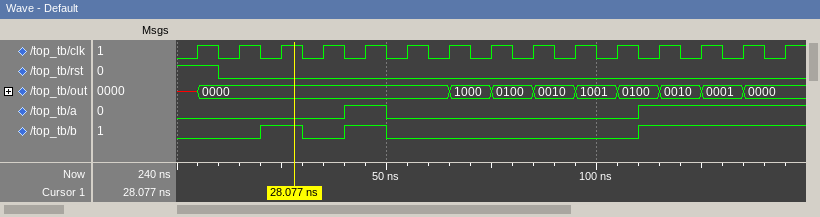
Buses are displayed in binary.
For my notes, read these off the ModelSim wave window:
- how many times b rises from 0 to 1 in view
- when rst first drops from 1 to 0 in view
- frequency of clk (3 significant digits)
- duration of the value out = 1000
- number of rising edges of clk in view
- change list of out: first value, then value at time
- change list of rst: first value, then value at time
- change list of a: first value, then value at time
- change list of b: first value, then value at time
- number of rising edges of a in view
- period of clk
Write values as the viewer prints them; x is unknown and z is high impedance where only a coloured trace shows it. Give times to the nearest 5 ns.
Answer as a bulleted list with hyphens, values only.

- 3
- 10 ns
- 100 MHz
- 10 ns
- 15
- x, 0000 at 5 ns, 1000 at 65 ns, 0100 at 75 ns, 0010 at 85 ns, 1001 at 95 ns, 0100 at 105 ns, 0010 at 115 ns, 0001 at 125 ns, 0000 at 135 ns
- 1, 0 at 10 ns
- 0, 1 at 40 ns, 0 at 50 ns, 1 at 110 ns
- 0, 1 at 20 ns, 0 at 30 ns, 1 at 40 ns, 0 at 50 ns, 1 at 110 ns
- 2
- 10 ns
